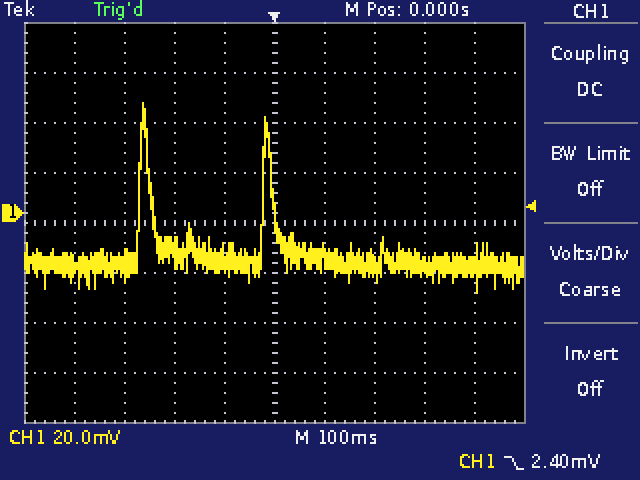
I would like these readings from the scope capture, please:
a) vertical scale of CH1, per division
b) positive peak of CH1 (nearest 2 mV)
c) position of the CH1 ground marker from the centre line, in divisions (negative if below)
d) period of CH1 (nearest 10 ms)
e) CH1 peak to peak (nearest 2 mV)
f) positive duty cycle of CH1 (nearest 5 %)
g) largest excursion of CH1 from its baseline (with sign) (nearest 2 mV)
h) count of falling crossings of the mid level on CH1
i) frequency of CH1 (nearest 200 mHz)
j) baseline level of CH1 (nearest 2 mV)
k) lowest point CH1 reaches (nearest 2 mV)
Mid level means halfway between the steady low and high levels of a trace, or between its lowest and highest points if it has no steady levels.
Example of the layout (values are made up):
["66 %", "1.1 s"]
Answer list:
["20 mV", "44 mV", "+0.2 div", "250 ms", "76 mV", "10 %", "+64 mV", "2", "4.0 Hz", "-20 mV", "-32 mV"]
